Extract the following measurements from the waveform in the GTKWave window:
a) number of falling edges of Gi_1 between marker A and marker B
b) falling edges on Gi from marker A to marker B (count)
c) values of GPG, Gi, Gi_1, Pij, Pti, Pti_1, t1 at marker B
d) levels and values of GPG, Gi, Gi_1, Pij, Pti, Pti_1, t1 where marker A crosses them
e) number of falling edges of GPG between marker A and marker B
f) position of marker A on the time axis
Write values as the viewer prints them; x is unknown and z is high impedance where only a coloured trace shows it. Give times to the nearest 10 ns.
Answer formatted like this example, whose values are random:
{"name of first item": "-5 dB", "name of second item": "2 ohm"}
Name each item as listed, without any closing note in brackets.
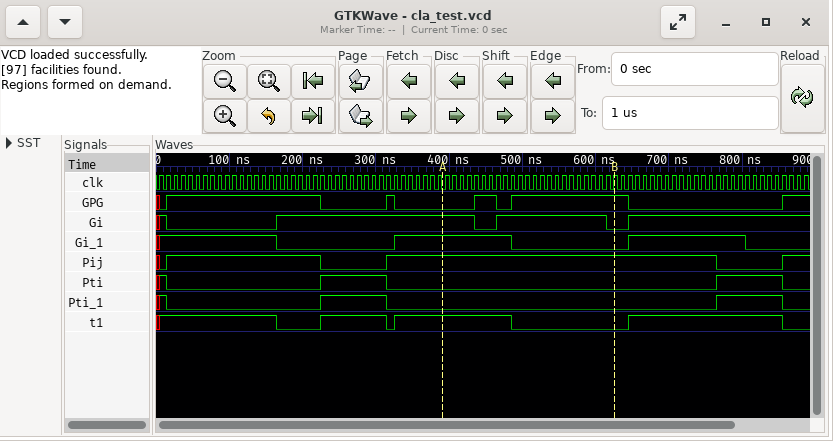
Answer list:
{"number of falling edges of Gi_1 between marker A and marker B": "1", "falling edges on Gi from marker A to marker B": "2", "values of GPG, Gi, Gi_1, Pij, Pti, Pti_1, t1 at marker B": "GPG=1, Gi=0, Gi_1=0, Pij=1, Pti=0, Pti_1=0, t1=0", "levels and values of GPG, Gi, Gi_1, Pij, Pti, Pti_1, t1 where marker A crosses them": "GPG=0, Gi=1, Gi_1=1, Pij=1, Pti=0, Pti_1=0, t1=1", "number of falling edges of GPG between marker A and marker B": "1", "position of marker A on the time axis": "390 ns"}
